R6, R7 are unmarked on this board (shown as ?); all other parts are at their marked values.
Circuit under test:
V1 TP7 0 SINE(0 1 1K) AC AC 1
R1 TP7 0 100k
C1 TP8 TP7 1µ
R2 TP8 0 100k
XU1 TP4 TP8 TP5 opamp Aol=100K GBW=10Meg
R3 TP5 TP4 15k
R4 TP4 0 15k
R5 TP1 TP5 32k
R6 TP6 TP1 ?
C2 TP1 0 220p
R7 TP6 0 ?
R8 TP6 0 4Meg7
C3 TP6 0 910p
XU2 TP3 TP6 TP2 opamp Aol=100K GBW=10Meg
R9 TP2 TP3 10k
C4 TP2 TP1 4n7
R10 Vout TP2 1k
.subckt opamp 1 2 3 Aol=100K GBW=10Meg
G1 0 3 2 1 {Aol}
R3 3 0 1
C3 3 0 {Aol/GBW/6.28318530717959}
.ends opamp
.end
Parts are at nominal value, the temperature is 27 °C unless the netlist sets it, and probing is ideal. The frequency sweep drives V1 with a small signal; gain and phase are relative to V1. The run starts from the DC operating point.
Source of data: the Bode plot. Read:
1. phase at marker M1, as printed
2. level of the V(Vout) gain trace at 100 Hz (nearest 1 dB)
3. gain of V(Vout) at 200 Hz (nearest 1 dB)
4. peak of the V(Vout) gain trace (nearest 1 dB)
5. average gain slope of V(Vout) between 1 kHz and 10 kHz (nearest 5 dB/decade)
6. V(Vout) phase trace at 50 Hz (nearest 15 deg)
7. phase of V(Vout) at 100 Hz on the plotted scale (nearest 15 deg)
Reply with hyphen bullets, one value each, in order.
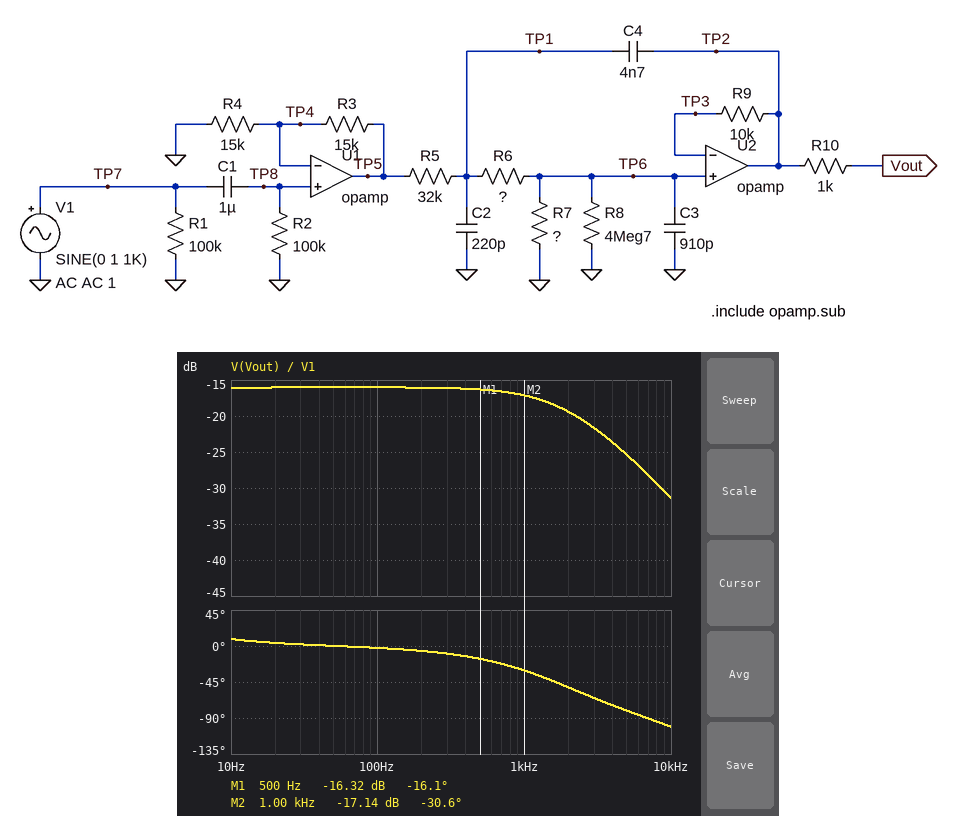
- -16.1 deg
- -16 dB
- -16 dB
- -16 dB
- -15 dB/decade
- 0 deg
- 0 deg
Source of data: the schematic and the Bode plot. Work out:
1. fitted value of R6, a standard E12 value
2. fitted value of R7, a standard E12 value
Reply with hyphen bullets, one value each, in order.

- 47 kΩ
- 6.8 kΩ
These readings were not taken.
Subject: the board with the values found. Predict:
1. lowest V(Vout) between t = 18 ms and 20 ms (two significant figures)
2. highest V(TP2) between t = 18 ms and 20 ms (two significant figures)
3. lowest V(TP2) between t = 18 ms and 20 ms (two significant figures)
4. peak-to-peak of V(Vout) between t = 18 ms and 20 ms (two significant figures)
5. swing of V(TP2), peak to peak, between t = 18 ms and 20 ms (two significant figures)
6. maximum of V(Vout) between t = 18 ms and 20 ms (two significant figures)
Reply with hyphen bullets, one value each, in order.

- -140 mV
- 140 mV
- -140 mV
- 280 mV
- 280 mV
- 140 mV
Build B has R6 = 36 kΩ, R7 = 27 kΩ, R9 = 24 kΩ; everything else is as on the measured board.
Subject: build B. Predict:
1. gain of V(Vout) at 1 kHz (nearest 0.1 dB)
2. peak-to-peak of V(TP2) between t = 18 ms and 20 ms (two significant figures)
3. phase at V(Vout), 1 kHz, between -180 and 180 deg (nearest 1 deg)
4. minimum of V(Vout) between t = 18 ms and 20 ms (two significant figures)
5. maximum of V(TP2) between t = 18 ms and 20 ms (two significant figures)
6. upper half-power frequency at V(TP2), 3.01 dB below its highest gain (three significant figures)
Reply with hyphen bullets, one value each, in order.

- -5.5 dB
- 1.1 V
- -28 deg
- -530 mV
- 530 mV
- 2.55 kHz
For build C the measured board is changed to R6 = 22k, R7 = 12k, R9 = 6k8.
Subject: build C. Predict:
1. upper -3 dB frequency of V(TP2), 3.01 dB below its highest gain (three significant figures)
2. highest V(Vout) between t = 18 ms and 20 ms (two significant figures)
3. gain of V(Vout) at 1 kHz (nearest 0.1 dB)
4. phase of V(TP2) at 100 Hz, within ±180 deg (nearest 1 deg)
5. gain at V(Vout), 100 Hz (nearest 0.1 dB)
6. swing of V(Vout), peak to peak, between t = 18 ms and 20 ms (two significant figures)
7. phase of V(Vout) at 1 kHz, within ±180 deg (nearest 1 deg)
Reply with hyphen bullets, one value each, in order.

- 2.96 kHz
- 340 mV
- -9.3 dB
- -1 deg
- -8.8 dB
- 690 mV
- -22 deg
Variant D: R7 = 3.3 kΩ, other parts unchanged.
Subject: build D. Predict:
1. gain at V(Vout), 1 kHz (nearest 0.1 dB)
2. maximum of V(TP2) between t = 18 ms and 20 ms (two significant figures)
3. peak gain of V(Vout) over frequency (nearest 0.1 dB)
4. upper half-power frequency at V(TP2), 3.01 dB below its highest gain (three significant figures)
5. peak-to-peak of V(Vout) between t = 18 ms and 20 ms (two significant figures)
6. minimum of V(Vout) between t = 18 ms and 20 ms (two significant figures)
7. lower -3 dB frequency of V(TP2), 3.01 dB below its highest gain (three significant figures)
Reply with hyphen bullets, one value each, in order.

- -23.1 dB
- 70 mV
- -21.9 dB
- 1.77 kHz
- 140 mV
- -70 mV
- 1.59 Hz
